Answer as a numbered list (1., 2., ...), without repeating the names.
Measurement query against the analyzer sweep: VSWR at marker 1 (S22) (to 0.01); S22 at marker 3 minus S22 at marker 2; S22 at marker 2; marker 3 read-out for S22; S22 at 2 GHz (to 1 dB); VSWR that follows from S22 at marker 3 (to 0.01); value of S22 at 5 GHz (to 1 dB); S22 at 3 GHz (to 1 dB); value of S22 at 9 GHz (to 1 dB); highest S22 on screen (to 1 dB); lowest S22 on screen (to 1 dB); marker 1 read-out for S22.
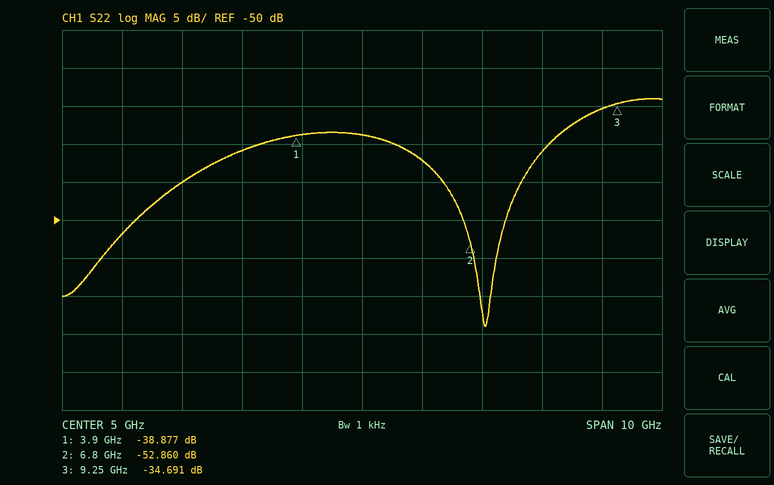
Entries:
1. 1.02
2. 18.169 dB
3. -52.860 dB
4. -34.691 dB
5. -45 dB
6. 1.04
7. -39 dB
8. -41 dB
9. -35 dB
10. -34 dB
11. -64 dB
12. -38.877 dB
